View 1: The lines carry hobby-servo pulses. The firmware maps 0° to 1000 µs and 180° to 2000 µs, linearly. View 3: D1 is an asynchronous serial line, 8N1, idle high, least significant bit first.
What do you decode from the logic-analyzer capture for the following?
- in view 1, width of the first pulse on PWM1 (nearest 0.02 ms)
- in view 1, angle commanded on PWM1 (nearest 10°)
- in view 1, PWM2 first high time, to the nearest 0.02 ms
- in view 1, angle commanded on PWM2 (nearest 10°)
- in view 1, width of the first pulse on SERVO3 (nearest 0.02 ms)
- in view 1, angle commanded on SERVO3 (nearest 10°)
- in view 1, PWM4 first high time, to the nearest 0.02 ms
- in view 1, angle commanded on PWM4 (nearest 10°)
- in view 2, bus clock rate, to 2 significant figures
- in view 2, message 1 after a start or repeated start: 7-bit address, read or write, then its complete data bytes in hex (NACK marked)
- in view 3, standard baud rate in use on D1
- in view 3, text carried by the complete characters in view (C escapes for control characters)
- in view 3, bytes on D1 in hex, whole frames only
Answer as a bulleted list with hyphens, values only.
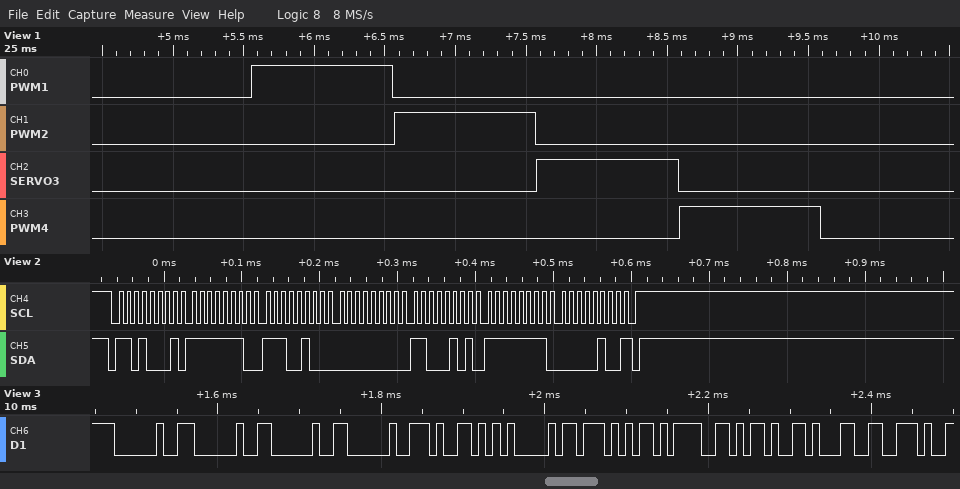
- 1.00 ms
- 0°
- 1.00 ms
- 0°
- 1.00 ms
- 0°
- 1.00 ms
- 0°
- 100 kHz
- 0x68 read: FE E4 00 C5 FF 04 NACK
- 115200 baud
- "    YAW=-1."
- 20 20 20 20 59 41 57 3D 2D 31 2E
